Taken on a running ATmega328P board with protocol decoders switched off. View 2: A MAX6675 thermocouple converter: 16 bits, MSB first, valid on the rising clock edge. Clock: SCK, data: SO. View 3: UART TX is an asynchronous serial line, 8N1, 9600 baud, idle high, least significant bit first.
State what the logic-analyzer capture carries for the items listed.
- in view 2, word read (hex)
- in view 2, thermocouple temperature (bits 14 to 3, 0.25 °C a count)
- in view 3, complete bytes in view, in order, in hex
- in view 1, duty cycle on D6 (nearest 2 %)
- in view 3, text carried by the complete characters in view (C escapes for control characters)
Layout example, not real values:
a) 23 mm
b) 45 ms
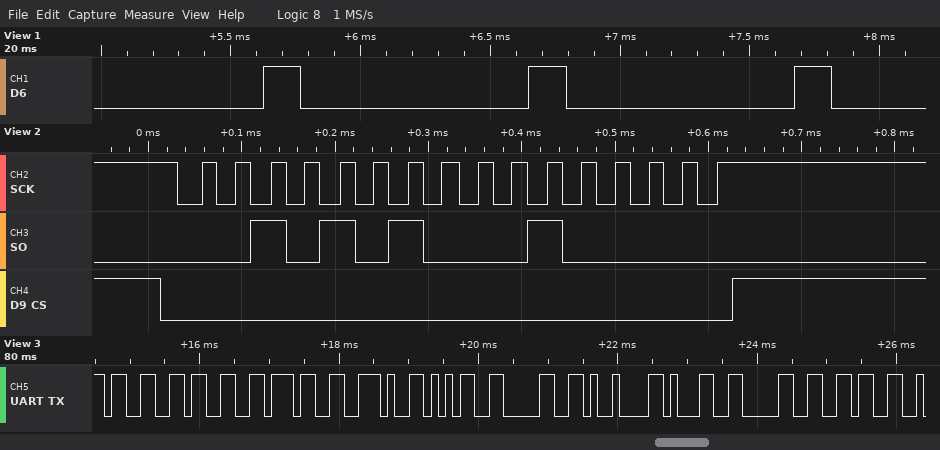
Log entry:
a) 0x2A20
b) 337.00 °C
c) 33 33 37 2E 35 30 09 31 30 36
d) 14 %
e) "337.50\t106"
